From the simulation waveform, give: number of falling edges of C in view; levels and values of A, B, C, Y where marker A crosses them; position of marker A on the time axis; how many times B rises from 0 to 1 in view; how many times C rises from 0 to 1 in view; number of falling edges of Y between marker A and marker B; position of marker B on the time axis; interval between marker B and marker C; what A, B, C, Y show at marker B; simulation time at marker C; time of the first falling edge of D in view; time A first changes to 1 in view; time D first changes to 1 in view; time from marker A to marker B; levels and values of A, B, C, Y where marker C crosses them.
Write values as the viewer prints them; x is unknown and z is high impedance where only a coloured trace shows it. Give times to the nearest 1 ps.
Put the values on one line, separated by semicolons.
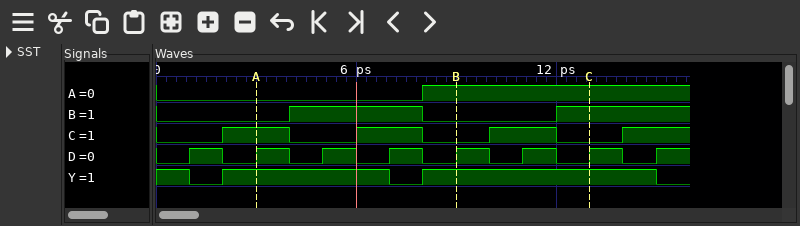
3; A=0, B=0, C=1, Y=1; 3 ps; 2; 4; 1; 9 ps; 4 ps; A=1, B=0, C=0, Y=1; 13 ps; 2 ps; 8 ps; 1 ps; 6 ps; A=1, B=1, C=0, Y=1
